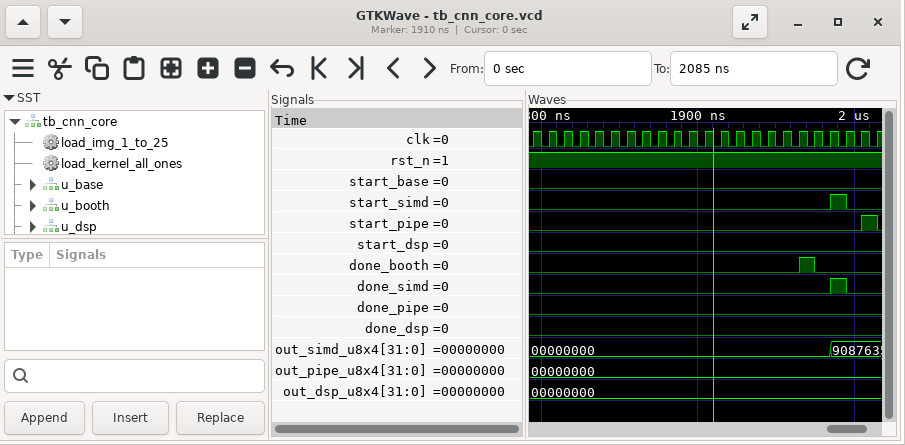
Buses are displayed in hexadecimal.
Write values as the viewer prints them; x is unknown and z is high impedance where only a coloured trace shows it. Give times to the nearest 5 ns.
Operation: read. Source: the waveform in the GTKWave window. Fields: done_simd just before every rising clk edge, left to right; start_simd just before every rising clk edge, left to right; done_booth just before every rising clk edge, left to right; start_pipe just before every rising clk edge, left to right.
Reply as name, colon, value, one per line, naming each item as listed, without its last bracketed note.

done_simd just before every rising clk edge, left to right: 0 0 0 0 0 0 0 0 0 0 0 0 0 0 0 0 0 0 0 0 1 0 0
start_simd just before every rising clk edge, left to right: 0 0 0 0 0 0 0 0 0 0 0 0 0 0 0 0 0 0 0 0 1 0 0
done_booth just before every rising clk edge, left to right: 0 0 0 0 0 0 0 0 0 0 0 0 0 0 0 0 0 0 1 0 0 0 0
start_pipe just before every rising clk edge, left to right: 0 0 0 0 0 0 0 0 0 0 0 0 0 0 0 0 0 0 0 0 0 0 1
